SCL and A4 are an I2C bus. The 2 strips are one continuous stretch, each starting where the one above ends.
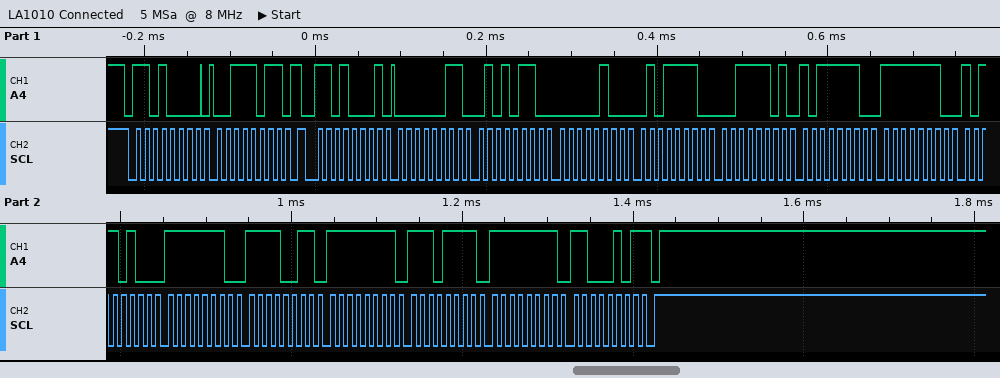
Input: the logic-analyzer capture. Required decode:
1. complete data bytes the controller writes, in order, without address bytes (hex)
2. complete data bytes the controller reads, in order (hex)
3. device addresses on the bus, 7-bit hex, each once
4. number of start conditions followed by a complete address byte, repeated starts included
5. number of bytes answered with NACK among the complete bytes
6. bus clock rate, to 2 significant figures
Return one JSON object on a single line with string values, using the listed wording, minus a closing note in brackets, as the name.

{"complete data bytes the controller writes, in order, without address bytes": "3B", "complete data bytes the controller reads, in order": "03 56 04 5E 3D BE FE B4 FE F3 FF EF FF C5", "device addresses on the bus, 7-bit hex, each once": "0x68", "number of start conditions followed by a complete address byte, repeated starts included": "2", "number of bytes answered with NACK among the complete bytes": "1", "bus clock rate, to 2 significant figures": "100 kHz"}
